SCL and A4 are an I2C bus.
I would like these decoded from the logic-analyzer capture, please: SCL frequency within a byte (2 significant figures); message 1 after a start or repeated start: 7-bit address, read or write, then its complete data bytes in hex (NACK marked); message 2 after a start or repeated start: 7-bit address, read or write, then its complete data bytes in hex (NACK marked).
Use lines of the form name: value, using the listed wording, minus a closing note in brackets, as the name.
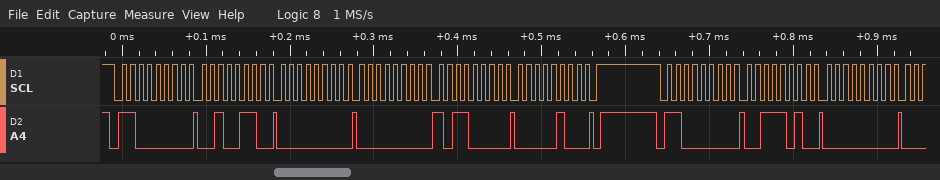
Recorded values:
SCL frequency within a byte: 100 kHz
message 1 after a start or repeated start: 7-bit address, read or write, then its complete data bytes in hex: 0x60 write: 26 00 00 B0 04
message 2 after a start or repeated start: 7-bit address, read or write, then its complete data bytes in hex: 0x60 write: 3A 00
